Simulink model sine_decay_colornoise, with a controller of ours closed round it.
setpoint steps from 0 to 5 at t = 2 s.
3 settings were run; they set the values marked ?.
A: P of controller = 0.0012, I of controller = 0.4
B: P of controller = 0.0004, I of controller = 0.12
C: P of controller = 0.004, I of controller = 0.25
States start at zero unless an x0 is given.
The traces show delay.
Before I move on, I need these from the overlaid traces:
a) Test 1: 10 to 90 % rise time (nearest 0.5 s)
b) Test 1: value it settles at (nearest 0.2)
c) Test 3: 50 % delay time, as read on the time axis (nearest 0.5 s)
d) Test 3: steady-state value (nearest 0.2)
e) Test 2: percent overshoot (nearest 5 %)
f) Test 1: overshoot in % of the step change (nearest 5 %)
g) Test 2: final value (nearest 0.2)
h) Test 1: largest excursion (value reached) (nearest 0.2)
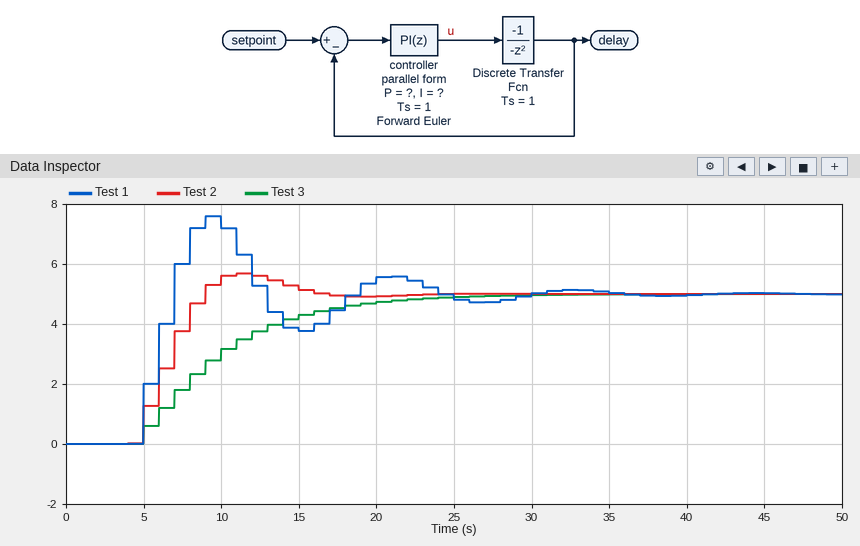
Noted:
2.0 s
5.0
9.0 s
5.0
15 %
50 %
5.0
7.6
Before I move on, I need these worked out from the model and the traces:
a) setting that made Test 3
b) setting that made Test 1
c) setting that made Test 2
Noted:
B
A
C
